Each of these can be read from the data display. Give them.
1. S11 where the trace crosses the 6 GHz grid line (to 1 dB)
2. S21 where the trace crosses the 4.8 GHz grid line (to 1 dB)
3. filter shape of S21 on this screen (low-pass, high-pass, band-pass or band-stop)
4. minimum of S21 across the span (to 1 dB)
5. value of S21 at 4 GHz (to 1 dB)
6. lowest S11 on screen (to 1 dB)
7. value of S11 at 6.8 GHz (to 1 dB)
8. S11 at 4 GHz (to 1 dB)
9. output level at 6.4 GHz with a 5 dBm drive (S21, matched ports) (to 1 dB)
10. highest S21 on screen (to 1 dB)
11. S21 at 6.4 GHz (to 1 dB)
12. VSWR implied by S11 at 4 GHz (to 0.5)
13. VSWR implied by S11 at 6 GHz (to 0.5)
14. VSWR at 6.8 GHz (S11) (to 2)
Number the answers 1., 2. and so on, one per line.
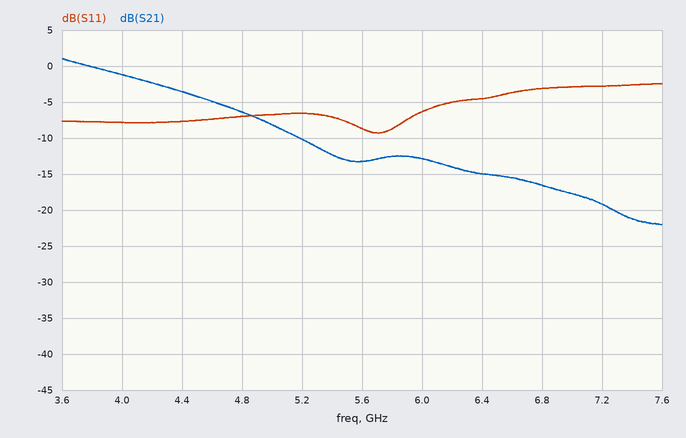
1. -6 dB
2. -6 dB
3. low-pass
4. -22 dB
5. -1 dB
6. -9 dB
7. -3 dB
8. -8 dB
9. -10 dBm
10. 1 dB
11. -15 dB
12. 2.5
13. 3.0
14. 6
